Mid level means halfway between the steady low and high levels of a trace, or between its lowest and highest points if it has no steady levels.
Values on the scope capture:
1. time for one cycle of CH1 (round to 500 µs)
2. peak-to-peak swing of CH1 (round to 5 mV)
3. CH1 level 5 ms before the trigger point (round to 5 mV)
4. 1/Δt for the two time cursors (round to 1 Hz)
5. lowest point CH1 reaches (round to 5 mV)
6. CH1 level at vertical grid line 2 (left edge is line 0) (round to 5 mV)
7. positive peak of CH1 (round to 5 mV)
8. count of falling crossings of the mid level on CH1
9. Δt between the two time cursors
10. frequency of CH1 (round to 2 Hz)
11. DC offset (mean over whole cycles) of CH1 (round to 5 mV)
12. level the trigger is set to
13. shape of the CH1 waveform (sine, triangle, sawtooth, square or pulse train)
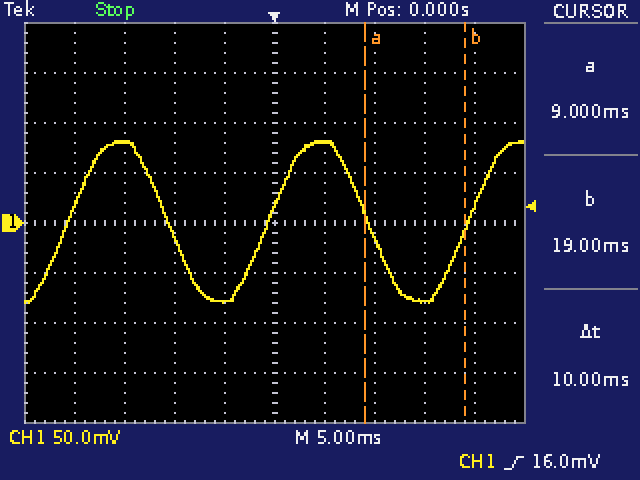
20.0 ms
160 mV
-80 mV
100 Hz
-80 mV
80 mV
80 mV
2
10 ms
50 Hz
0 mV
16.0 mV
sine
